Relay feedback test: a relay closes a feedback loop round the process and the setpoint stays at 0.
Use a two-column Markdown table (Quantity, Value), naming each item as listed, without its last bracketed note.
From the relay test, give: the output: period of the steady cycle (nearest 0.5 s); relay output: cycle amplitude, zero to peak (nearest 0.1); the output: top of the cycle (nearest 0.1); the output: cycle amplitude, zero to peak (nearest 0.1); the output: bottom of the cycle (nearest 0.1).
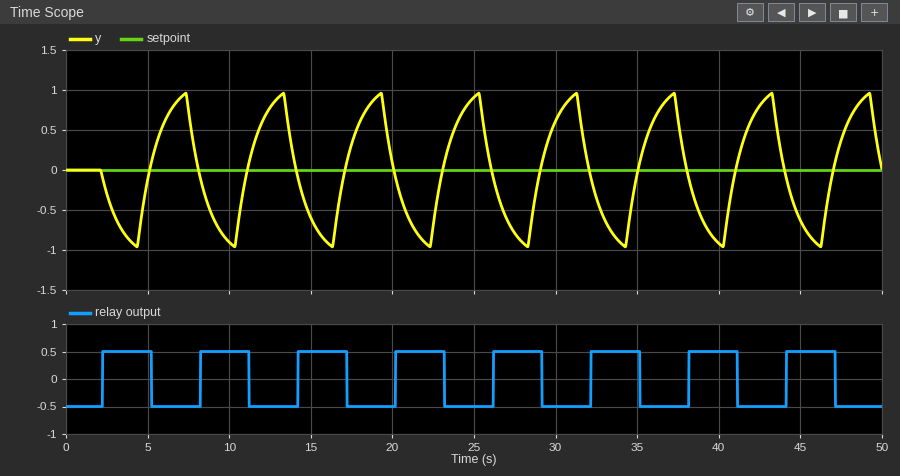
| Quantity | Value |
|---|---|
| the output: period of the steady cycle | 6.0 s |
| relay output: cycle amplitude, zero to peak | 0.5 |
| the output: top of the cycle | 1.0 |
| the output: cycle amplitude, zero to peak | 1.0 |
| the output: bottom of the cycle | -1.0 |
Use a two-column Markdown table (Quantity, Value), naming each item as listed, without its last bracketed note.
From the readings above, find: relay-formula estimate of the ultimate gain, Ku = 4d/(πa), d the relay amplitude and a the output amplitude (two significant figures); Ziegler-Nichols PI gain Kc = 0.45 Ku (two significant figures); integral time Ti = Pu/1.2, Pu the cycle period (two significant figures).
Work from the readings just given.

| Quantity | Value |
|---|---|
| relay-formula estimate of the ultimate gain, Ku = 4d/(πa), d the relay amplitude and a the output amplitude | 0.64 |
| Ziegler-Nichols PI gain Kc = 0.45 Ku | 0.29 |
| integral time Ti = Pu/1.2, Pu the cycle period | 5.0 s |
